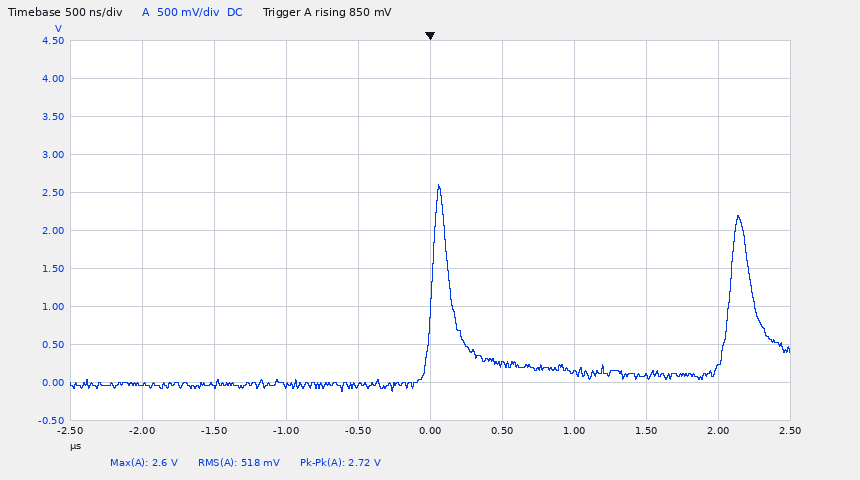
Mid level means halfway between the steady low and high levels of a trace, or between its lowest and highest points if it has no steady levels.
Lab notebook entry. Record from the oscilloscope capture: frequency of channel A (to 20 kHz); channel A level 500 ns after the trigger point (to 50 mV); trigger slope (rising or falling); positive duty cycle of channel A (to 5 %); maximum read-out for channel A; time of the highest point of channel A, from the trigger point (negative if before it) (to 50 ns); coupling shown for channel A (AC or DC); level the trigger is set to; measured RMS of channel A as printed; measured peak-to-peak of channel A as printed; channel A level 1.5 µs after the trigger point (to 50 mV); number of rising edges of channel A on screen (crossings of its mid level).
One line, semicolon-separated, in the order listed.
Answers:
480 kHz; 250 mV; rising; 5 %; 2.6 V; +50 ns; DC; 850 mV; 518 mV; 2.72 V; 100 mV; 2
